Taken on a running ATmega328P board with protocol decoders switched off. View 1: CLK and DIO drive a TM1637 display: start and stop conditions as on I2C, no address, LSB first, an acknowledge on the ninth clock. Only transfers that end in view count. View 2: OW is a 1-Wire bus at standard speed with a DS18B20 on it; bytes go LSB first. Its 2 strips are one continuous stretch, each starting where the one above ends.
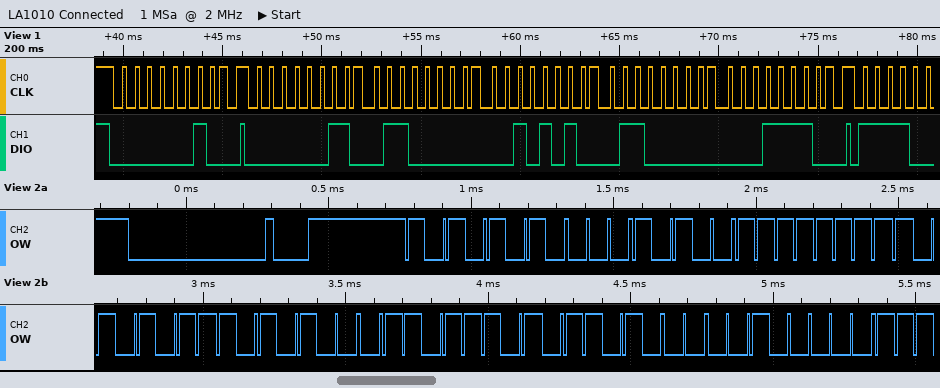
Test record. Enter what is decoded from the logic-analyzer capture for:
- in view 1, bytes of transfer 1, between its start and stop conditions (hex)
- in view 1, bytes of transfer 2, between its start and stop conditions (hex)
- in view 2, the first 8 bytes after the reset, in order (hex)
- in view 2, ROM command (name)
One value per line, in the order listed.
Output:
40
C0 06 54 06 78
55 28 FF D5 15 BB 16 04
Match ROM
